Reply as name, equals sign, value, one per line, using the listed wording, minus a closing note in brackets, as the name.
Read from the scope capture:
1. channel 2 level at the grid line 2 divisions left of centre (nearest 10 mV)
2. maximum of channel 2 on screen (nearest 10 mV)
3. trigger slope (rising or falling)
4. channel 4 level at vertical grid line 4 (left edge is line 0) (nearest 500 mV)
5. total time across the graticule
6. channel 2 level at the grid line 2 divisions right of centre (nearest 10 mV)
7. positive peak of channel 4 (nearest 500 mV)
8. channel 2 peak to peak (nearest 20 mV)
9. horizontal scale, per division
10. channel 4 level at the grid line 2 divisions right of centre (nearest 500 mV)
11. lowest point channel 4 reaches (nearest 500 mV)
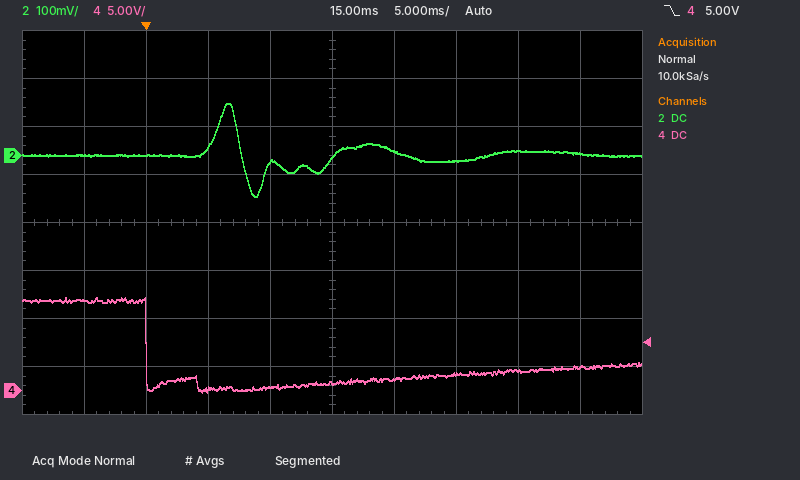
channel 2 level at the grid line 2 divisions left of centre = 20 mV
maximum of channel 2 on screen = 110 mV
trigger slope = falling
channel 4 level at vertical grid line 4 (left edge is line 0) = 500 mV
total time across the graticule = 50 ms
channel 2 level at the grid line 2 divisions right of centre = -10 mV
positive peak of channel 4 = 9.5 V
channel 2 peak to peak = 200 mV
horizontal scale, per division = 5 ms
channel 4 level at the grid line 2 divisions right of centre = 1.5 V
lowest point channel 4 reaches = 0.0 V
